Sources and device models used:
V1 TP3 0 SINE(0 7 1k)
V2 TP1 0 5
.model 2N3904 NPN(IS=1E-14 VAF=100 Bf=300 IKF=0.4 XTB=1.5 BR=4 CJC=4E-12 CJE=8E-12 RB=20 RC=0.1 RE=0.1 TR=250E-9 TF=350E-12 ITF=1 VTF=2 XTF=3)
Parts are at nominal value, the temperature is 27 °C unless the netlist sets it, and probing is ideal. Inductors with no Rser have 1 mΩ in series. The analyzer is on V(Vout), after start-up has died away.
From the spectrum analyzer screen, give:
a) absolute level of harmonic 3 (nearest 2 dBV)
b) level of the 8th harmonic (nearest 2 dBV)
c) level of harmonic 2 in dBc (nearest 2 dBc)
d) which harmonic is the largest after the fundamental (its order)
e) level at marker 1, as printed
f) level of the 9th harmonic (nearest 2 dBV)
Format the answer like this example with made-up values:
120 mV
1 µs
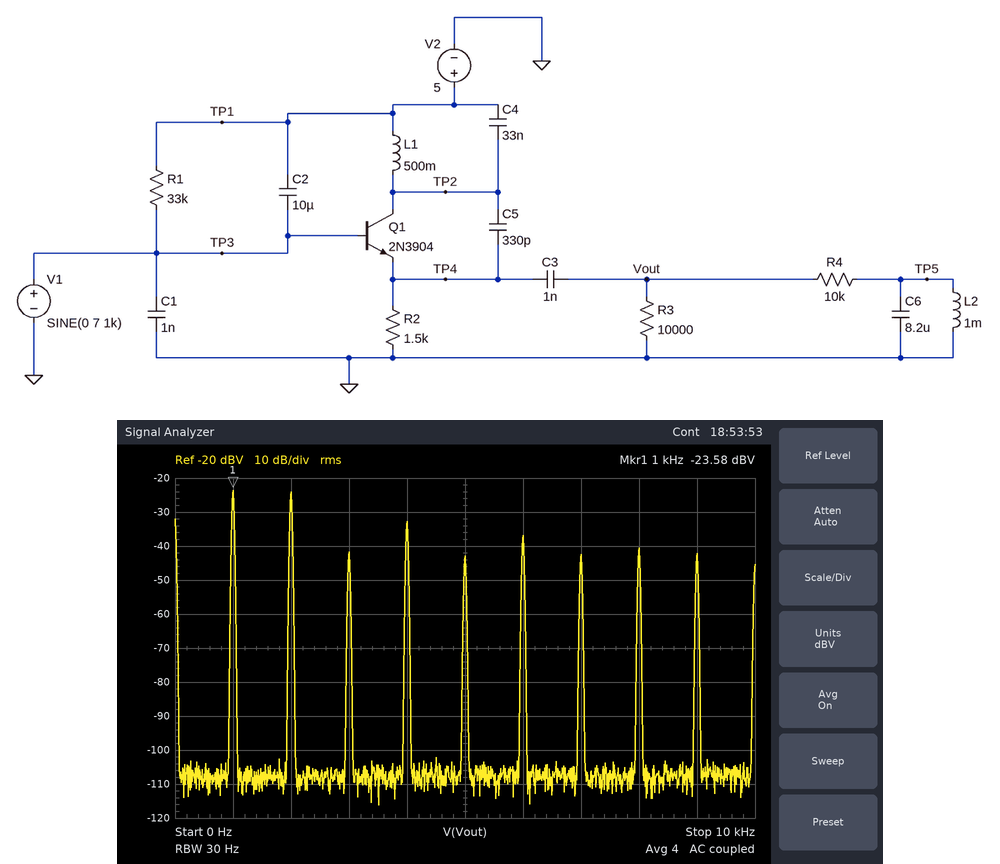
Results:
-42 dBV
-40 dBV
0 dBc
2
-23.58 dBV
-42 dBV
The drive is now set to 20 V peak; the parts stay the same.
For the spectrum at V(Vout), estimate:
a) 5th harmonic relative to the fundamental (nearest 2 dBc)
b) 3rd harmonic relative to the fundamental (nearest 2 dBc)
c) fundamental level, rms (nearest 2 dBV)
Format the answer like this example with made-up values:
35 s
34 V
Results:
-24 dBc
-24 dBc
-14 dBV
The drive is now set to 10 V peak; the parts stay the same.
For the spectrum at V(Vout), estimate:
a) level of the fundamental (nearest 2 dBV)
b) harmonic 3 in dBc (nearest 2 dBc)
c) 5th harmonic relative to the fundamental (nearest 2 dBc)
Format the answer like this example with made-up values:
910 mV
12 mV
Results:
-20 dBV
-22 dBc
-22 dBc
